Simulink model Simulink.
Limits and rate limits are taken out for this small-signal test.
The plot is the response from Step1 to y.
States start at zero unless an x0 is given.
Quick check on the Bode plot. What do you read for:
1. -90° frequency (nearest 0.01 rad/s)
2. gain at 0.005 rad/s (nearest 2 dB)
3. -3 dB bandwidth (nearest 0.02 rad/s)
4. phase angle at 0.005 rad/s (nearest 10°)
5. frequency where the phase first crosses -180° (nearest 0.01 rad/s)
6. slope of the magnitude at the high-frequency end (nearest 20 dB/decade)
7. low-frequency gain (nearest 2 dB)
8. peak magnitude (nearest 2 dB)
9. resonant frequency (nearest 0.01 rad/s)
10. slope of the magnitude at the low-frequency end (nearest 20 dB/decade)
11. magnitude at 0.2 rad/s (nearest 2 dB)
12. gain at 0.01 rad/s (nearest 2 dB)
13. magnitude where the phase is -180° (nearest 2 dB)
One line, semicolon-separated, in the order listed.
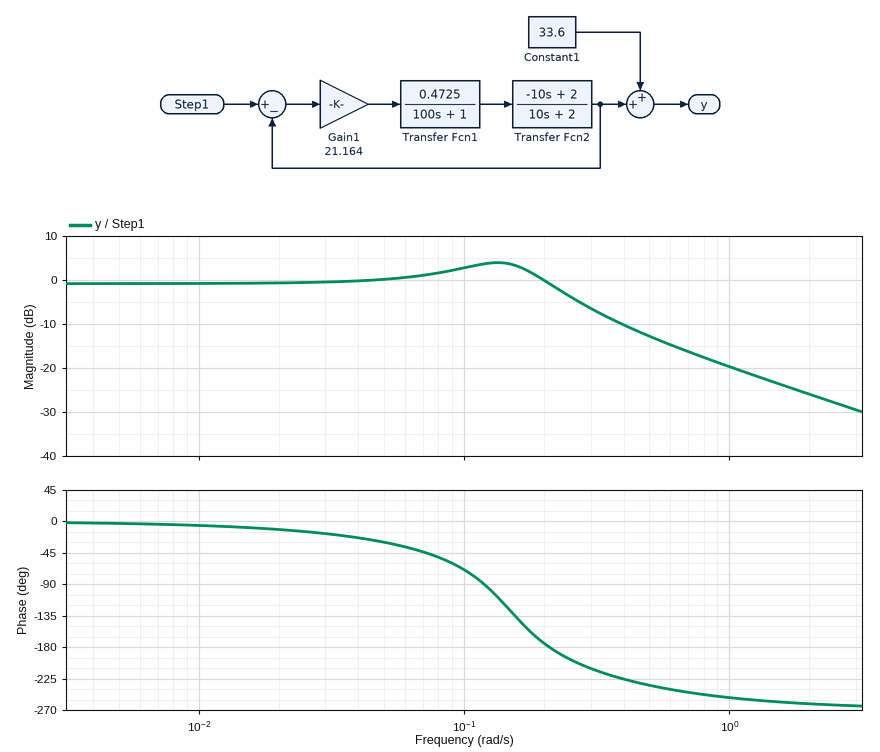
0.12 rad/s; 0 dB; 0.26 rad/s; 0°; 0.21 rad/s; -20 dB/decade; 0 dB; 4 dB; 0.13 rad/s; 0 dB/decade; 0 dB; 0 dB; 0 dB
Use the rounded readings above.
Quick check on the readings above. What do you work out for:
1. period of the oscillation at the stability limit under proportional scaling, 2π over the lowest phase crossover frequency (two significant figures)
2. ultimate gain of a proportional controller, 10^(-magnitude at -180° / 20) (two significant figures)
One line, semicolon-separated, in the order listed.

30 s; 1.0
